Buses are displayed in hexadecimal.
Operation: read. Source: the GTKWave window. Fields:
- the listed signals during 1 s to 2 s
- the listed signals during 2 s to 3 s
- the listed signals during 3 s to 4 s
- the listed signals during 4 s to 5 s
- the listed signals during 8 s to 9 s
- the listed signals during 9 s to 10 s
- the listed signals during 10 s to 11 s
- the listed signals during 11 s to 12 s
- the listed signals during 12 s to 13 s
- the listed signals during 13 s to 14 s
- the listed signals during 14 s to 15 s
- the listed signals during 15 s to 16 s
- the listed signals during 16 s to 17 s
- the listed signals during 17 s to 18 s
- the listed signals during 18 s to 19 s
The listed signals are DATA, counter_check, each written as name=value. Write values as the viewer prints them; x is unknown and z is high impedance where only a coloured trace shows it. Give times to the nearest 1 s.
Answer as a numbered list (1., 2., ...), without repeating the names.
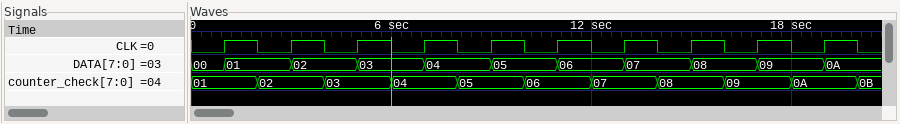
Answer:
1. DATA=01, counter_check=01
2. DATA=01, counter_check=02
3. DATA=02, counter_check=02
4. DATA=02, counter_check=03
5. DATA=04, counter_check=05
6. DATA=05, counter_check=05
7. DATA=05, counter_check=06
8. DATA=06, counter_check=06
9. DATA=06, counter_check=07
10. DATA=07, counter_check=07
11. DATA=07, counter_check=08
12. DATA=08, counter_check=08
13. DATA=08, counter_check=09
14. DATA=09, counter_check=09
15. DATA=09, counter_check=0A
